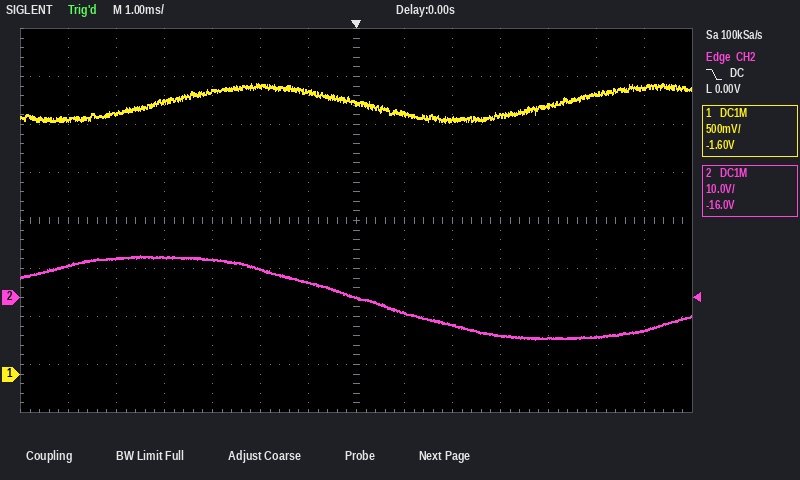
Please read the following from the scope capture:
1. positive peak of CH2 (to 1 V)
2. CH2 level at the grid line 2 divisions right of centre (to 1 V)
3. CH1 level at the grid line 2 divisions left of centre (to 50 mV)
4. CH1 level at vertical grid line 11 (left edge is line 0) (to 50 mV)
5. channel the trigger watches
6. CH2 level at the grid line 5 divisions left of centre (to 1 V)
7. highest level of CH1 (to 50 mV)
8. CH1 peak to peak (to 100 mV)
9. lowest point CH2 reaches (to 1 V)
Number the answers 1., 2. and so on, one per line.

1. 9 V
2. -6 V
3. 3.00 V
4. 2.80 V
5. CH2
6. 8 V
7. 3.05 V
8. 400 mV
9. -9 V
